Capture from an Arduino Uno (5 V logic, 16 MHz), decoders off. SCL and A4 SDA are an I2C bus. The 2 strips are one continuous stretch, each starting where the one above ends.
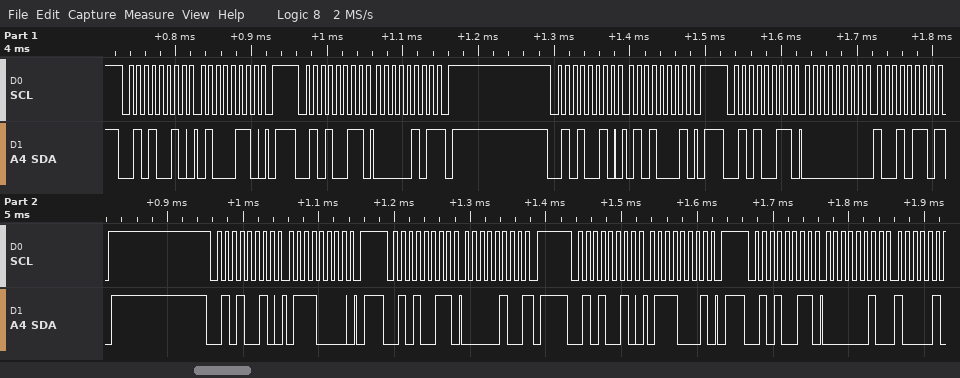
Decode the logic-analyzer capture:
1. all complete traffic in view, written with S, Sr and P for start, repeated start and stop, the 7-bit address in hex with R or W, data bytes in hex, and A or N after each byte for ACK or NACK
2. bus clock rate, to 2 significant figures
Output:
S 29W A 46 A P S 29R A 05 N P S 29W A 51 A P S 29R A 00 A 96 N P S 29W A 70 A P S 29R A 04 N P S 29W A 71 A P S 29R A 02 A
100 kHz
